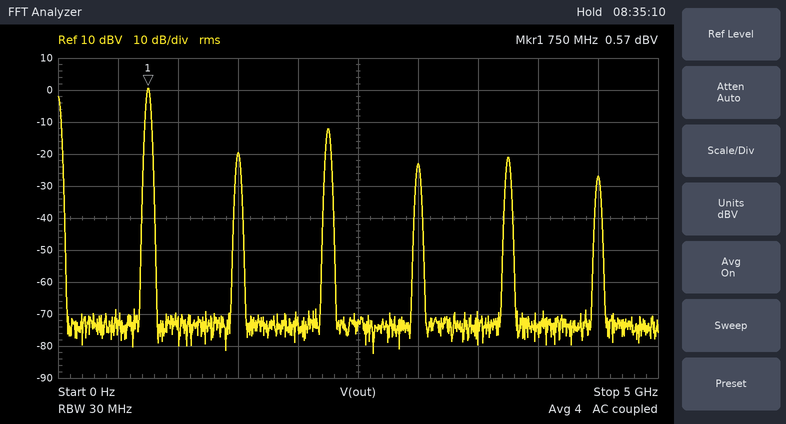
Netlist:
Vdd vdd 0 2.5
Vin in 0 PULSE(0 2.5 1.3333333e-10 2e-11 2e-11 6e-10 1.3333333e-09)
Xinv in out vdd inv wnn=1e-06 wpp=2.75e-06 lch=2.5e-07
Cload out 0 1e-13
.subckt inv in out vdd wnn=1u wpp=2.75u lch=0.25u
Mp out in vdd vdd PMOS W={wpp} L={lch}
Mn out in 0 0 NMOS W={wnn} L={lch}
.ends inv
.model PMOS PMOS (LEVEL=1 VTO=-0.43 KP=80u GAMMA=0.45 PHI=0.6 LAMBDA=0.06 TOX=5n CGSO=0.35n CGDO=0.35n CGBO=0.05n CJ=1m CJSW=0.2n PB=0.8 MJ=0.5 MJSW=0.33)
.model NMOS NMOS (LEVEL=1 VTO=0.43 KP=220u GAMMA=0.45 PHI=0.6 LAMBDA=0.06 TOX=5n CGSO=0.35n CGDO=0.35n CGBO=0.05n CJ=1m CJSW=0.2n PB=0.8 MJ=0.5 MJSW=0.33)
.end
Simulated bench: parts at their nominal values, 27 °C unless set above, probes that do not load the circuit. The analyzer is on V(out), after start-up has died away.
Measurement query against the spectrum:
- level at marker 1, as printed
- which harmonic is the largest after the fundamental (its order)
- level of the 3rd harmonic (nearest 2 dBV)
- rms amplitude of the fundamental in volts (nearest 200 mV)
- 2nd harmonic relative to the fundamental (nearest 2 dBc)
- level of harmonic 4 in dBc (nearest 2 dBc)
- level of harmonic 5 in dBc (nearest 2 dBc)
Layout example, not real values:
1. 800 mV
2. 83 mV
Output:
1. 0.57 dBV
2. 3
3. -12 dBV
4. 1.0 V
5. -20 dBc
6. -24 dBc
7. -22 dBc
